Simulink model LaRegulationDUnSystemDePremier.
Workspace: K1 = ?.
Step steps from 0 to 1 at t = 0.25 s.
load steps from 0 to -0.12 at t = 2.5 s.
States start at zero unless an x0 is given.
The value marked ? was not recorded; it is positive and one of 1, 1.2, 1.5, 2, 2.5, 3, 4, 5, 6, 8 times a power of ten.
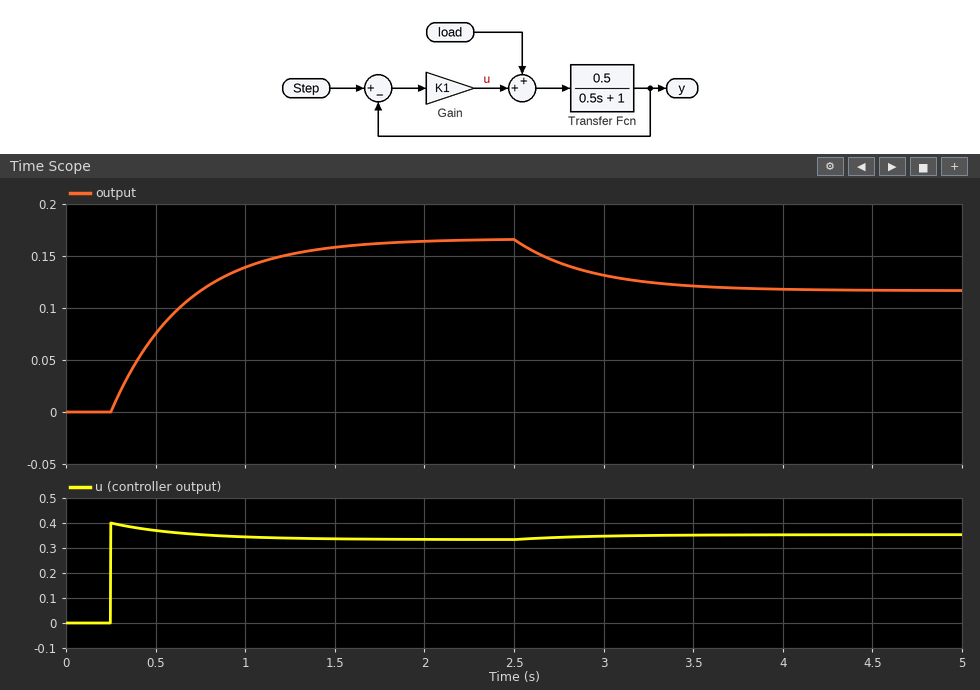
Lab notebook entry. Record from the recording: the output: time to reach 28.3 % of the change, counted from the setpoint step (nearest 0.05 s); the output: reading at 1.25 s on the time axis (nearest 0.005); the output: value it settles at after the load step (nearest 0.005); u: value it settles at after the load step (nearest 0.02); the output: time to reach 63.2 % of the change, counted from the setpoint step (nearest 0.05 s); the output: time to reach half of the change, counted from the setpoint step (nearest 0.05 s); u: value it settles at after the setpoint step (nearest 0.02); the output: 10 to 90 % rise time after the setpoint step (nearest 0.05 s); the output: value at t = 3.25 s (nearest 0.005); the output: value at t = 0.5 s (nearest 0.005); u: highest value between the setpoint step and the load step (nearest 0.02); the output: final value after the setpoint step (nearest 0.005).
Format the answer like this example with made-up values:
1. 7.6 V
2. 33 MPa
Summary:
1. 0.15 s
2. 0.150
3. 0.115
4. 0.36
5. 0.40 s
6. 0.30 s
7. 0.34
8. 0.90 s
9. 0.125
10. 0.075
11. 0.40
12. 0.165
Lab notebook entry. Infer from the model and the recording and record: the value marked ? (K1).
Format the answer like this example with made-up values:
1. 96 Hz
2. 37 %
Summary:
1. 0.4
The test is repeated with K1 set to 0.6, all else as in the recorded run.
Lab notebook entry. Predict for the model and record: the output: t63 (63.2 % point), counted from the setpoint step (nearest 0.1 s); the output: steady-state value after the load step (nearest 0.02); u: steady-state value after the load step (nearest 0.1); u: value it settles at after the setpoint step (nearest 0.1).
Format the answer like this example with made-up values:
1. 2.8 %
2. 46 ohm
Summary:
1. 0.4 s
2. 0.18
3. 0.5
4. 0.5
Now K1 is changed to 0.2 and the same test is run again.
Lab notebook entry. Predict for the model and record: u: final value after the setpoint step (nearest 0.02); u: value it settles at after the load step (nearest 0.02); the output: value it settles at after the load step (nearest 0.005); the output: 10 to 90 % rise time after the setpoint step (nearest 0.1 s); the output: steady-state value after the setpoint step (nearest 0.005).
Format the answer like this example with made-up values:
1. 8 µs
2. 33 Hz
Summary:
1. 0.18
2. 0.20
3. 0.035
4. 1.0 s
5. 0.090
